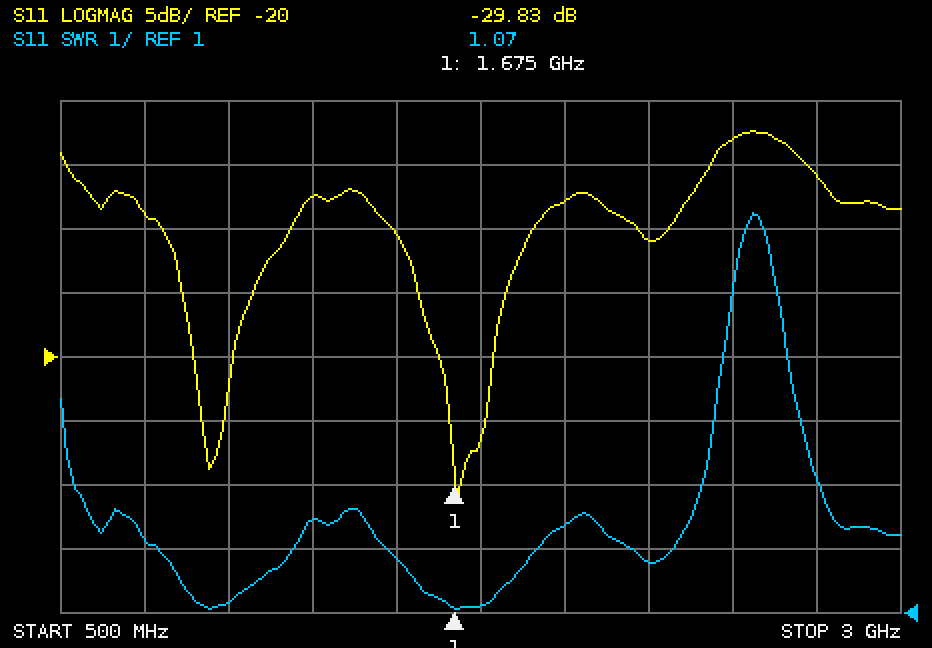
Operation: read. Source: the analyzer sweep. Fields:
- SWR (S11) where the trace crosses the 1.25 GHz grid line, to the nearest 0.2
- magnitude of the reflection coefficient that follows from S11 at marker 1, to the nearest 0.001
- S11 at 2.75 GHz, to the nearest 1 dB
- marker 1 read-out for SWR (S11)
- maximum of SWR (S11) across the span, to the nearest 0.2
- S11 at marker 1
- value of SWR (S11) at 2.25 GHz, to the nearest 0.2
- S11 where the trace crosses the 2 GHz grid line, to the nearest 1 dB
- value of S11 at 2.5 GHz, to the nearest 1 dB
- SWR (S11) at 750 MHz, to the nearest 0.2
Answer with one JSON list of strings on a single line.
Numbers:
["2.4", "0.032", "-6 dB", "1.07", "7.2", "-29.83 dB", "1.8", "-8 dB", "-3 dB", "2.2"]
